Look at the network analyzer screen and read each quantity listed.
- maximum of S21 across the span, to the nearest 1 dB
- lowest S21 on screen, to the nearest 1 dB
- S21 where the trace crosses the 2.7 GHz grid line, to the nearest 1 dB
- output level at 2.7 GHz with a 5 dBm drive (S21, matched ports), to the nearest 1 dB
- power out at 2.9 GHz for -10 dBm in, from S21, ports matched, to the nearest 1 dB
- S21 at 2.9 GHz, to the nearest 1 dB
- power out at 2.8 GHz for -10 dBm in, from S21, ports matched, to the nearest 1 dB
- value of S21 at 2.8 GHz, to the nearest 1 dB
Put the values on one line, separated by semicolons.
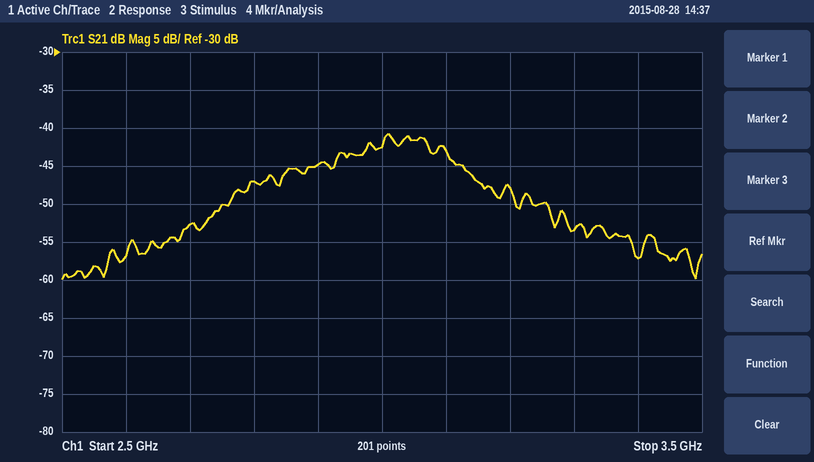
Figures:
-41 dB; -60 dB; -53 dB; -48 dBm; -55 dBm; -45 dB; -57 dBm; -47 dB
